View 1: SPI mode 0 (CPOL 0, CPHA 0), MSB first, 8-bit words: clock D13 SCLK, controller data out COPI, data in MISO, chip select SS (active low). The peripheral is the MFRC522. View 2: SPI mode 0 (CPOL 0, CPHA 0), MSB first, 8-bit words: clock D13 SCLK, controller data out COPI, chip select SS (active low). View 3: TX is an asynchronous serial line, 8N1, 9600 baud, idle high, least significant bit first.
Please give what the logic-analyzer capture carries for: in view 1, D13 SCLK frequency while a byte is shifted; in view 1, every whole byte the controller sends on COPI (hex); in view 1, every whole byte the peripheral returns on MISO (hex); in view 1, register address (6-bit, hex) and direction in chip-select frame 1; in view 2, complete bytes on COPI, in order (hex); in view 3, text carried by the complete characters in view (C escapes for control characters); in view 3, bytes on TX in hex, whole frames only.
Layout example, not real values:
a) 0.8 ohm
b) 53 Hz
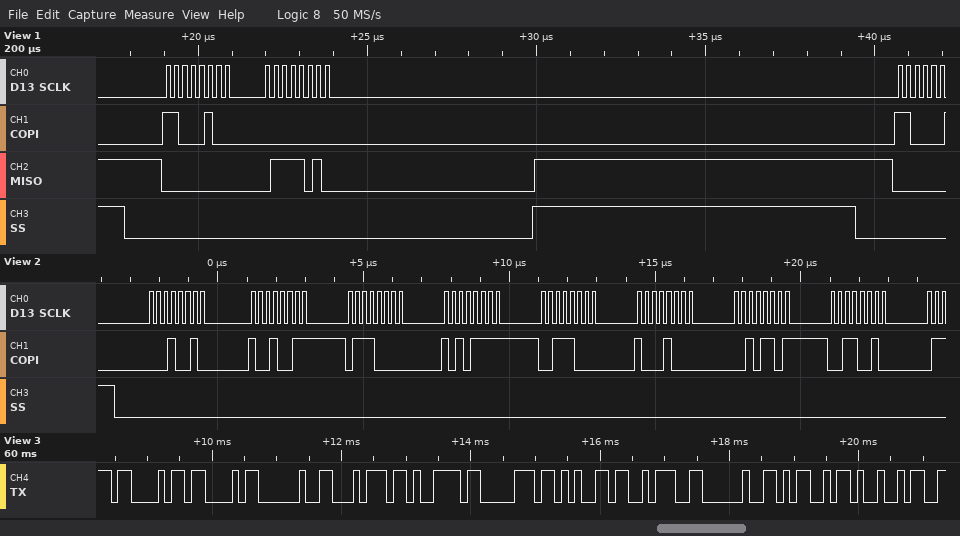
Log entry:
a) 4 MHz
b) C4 00
c) 00 7A
d) 0x22 read
e) 12 93 70 AF 38 88 2D 32
f) "CC type: MI"
g) 43 43 20 74 79 70 65 3A 20 4D 49
